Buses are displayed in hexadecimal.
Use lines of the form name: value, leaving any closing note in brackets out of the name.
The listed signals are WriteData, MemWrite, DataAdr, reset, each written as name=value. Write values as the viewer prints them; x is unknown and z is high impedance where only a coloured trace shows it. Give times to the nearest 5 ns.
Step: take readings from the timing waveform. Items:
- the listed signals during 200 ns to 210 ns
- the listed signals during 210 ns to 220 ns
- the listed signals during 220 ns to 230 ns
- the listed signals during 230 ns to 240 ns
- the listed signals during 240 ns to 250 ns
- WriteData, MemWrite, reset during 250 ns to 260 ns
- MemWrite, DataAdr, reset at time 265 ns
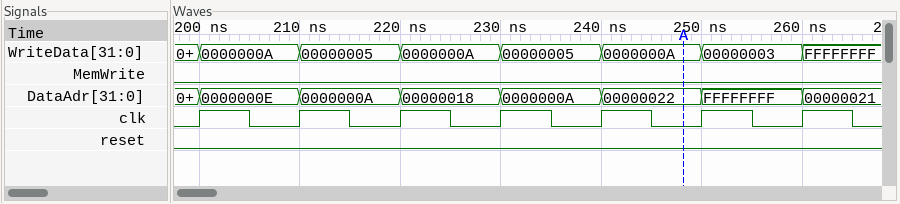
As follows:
the listed signals during 200 ns to 210 ns: WriteData=0000000A, MemWrite=0, DataAdr=0000000E, reset=0
the listed signals during 210 ns to 220 ns: WriteData=00000005, MemWrite=0, DataAdr=0000000A, reset=0
the listed signals during 220 ns to 230 ns: WriteData=0000000A, MemWrite=0, DataAdr=00000018, reset=0
the listed signals during 230 ns to 240 ns: WriteData=00000005, MemWrite=0, DataAdr=0000000A, reset=0
the listed signals during 240 ns to 250 ns: WriteData=0000000A, MemWrite=0, DataAdr=00000022, reset=0
WriteData, MemWrite, reset during 250 ns to 260 ns: WriteData=00000003, MemWrite=0, reset=0
MemWrite, DataAdr, reset at time 265 ns: MemWrite=0, DataAdr=00000021, reset=0
